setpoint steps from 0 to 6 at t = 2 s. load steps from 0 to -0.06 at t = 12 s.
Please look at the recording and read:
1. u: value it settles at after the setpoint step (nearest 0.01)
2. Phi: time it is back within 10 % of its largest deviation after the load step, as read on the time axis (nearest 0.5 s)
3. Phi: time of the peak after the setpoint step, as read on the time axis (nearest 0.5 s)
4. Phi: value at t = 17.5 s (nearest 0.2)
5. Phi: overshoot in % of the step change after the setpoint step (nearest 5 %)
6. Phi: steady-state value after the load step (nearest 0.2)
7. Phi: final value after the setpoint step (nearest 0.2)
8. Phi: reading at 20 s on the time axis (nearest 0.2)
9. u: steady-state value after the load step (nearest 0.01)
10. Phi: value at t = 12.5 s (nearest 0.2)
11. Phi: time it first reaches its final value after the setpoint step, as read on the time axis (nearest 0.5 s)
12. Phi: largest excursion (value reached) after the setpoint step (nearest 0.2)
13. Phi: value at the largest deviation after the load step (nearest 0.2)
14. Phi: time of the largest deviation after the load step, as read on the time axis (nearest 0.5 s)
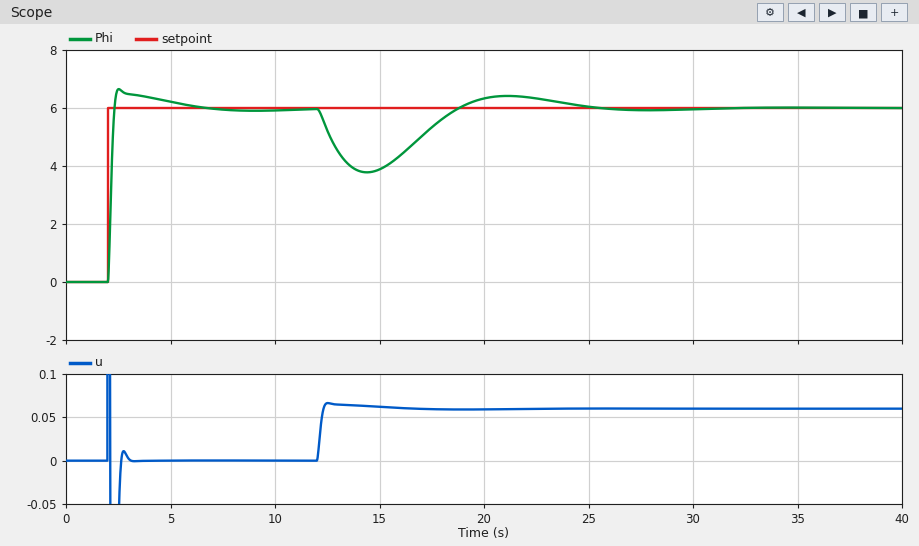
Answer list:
0.00
23.5 s
2.5 s
5.4
10 %
6.0
6.0
6.4
0.06
5.2
2.5 s
6.6
3.8
14.5 s
